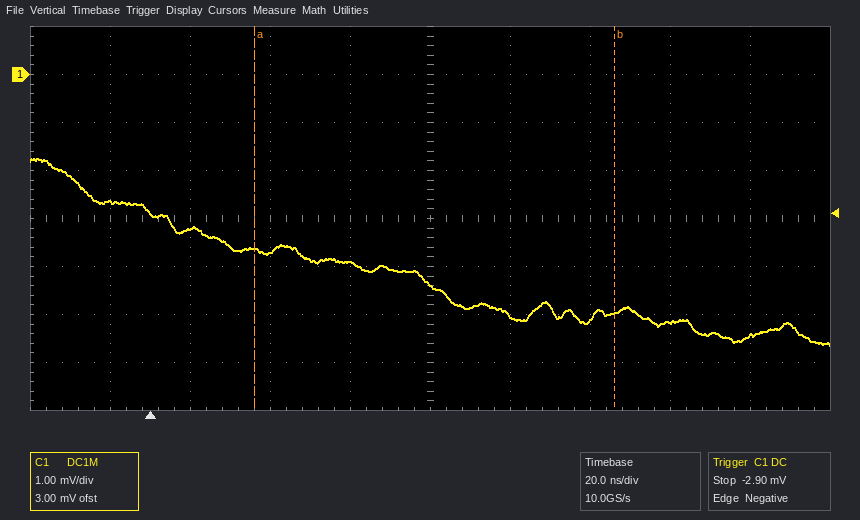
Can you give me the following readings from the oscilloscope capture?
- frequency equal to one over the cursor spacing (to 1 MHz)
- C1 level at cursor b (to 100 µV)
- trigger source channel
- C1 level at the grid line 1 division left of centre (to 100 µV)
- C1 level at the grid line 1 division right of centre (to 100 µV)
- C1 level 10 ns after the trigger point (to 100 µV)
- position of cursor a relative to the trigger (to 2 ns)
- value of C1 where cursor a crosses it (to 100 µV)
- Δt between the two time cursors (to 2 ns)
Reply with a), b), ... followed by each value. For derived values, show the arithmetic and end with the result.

a) 1 / 90 ns ≈ 11 MHz
b) -5.0 mV
c) C1
d) -3.9 mV
e) -5.0 mV
f) -3.2 mV
g) +26 ns
h) -3.6 mV
i) 90 ns
